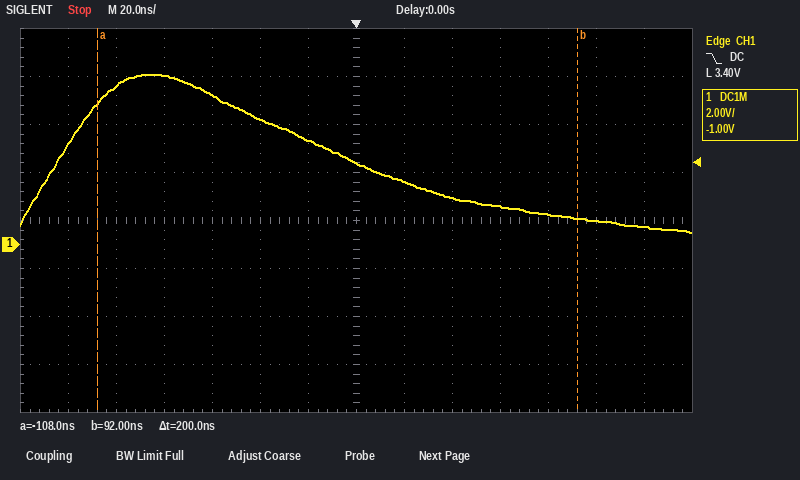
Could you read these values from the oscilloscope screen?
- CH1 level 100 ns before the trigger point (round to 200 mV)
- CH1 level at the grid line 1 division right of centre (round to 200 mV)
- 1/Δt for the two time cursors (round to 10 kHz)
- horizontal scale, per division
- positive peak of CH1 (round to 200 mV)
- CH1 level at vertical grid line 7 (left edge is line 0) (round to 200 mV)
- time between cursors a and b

6.6 V
2.6 V
5.00 MHz
20 ns
7.0 V
3.4 V
200 ns
